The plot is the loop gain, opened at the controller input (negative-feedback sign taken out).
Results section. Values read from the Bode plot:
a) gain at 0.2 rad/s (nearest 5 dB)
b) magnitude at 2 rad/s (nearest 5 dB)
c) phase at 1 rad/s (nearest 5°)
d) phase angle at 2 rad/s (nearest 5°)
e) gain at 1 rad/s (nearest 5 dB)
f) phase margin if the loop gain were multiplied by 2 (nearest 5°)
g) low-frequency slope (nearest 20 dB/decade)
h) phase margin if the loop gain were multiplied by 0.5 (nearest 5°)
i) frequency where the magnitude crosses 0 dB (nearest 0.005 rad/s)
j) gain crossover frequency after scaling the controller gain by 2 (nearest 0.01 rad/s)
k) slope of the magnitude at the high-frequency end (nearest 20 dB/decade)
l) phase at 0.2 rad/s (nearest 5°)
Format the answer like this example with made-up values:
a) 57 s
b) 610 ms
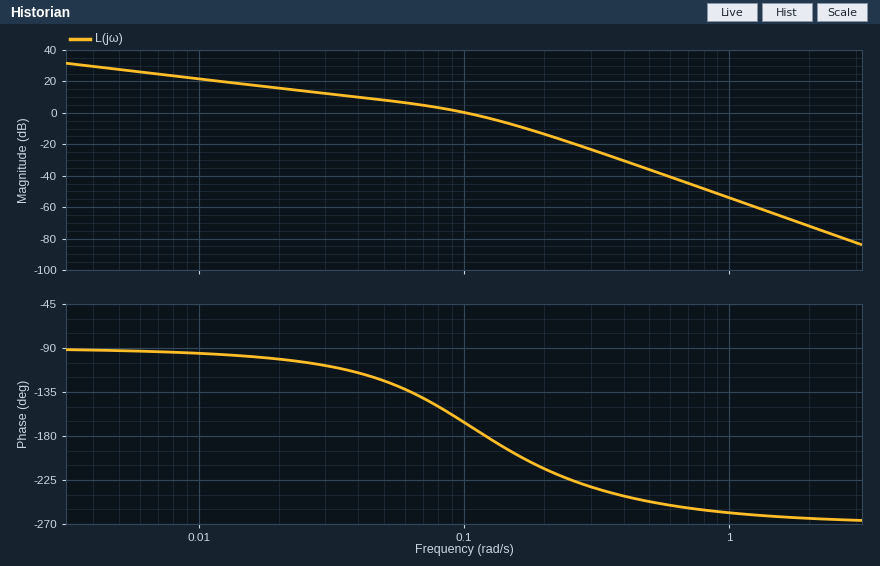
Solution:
a) -15 dB
b) -70 dB
c) -260°
d) -265°
e) -55 dB
f) -10°
g) -20 dB/decade
h) 45°
i) 0.100 rad/s
j) 0.14 rad/s
k) -60 dB/decade
l) -215°
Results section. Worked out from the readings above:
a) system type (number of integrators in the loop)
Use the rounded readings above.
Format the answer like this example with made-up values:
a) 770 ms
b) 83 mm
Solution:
a) 1
